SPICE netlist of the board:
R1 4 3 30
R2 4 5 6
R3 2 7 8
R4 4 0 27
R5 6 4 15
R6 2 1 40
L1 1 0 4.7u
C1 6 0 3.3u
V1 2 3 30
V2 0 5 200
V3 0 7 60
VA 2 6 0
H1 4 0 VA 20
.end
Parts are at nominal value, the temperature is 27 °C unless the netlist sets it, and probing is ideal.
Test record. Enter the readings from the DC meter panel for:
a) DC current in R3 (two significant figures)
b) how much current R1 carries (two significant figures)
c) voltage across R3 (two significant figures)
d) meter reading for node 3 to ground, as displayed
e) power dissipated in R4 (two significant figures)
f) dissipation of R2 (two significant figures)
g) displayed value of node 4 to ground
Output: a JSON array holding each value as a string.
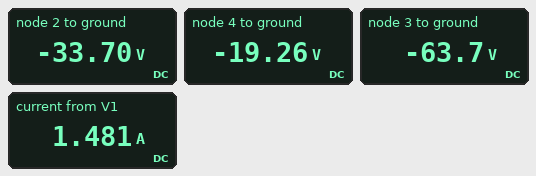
["3.3 A", "1.5 A", "26 V", "-63.7 V", "14 W", "5.4 kW", "-19.26 V"]
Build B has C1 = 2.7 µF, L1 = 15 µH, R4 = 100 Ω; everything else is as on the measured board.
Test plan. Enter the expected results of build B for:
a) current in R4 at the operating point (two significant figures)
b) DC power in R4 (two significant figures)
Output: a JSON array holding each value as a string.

["190 mA", "3.7 W"]
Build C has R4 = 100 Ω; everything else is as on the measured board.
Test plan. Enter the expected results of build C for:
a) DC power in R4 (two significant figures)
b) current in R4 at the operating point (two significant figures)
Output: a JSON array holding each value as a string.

["3.7 W", "190 mA"]
